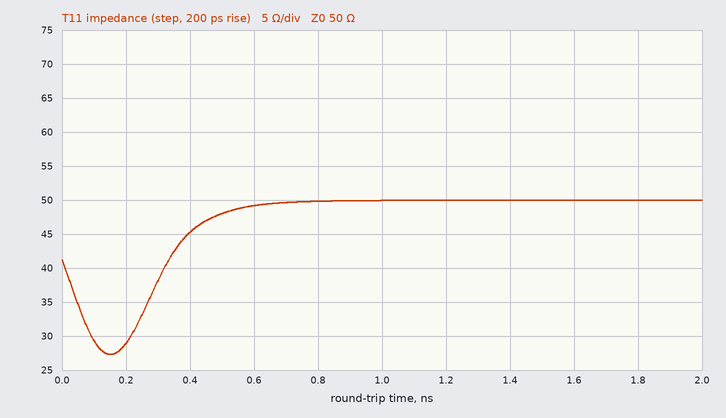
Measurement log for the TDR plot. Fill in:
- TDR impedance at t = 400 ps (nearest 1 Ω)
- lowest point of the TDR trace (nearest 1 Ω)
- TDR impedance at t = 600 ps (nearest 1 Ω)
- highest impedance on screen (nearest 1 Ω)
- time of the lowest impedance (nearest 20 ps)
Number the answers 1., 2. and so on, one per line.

1. 45 Ω
2. 27 Ω
3. 49 Ω
4. 50 Ω
5. 160 ps
